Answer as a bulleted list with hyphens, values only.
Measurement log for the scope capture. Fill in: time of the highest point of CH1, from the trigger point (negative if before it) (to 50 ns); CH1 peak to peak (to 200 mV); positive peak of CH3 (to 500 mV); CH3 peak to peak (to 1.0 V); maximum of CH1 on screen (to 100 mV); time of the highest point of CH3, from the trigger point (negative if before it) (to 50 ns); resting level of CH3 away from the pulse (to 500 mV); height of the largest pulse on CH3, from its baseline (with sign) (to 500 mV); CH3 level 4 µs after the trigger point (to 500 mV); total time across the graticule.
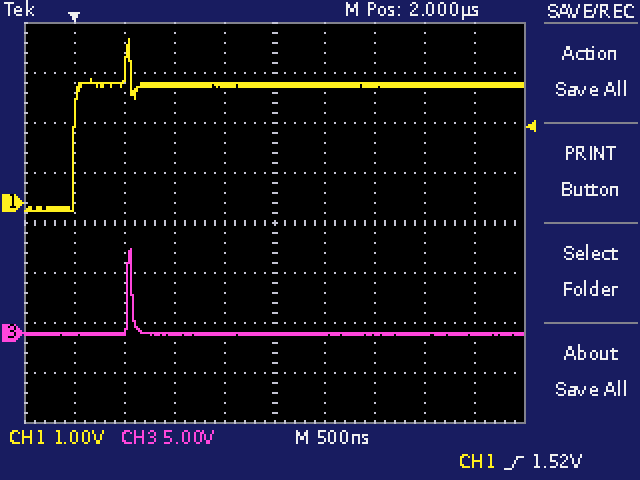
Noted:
- +550 ns
- 3.4 V
- 8.5 V
- 9.0 V
- 3.3 V
- +550 ns
- 0.0 V
- +8.5 V
- 0.0 V
- 5 µs
